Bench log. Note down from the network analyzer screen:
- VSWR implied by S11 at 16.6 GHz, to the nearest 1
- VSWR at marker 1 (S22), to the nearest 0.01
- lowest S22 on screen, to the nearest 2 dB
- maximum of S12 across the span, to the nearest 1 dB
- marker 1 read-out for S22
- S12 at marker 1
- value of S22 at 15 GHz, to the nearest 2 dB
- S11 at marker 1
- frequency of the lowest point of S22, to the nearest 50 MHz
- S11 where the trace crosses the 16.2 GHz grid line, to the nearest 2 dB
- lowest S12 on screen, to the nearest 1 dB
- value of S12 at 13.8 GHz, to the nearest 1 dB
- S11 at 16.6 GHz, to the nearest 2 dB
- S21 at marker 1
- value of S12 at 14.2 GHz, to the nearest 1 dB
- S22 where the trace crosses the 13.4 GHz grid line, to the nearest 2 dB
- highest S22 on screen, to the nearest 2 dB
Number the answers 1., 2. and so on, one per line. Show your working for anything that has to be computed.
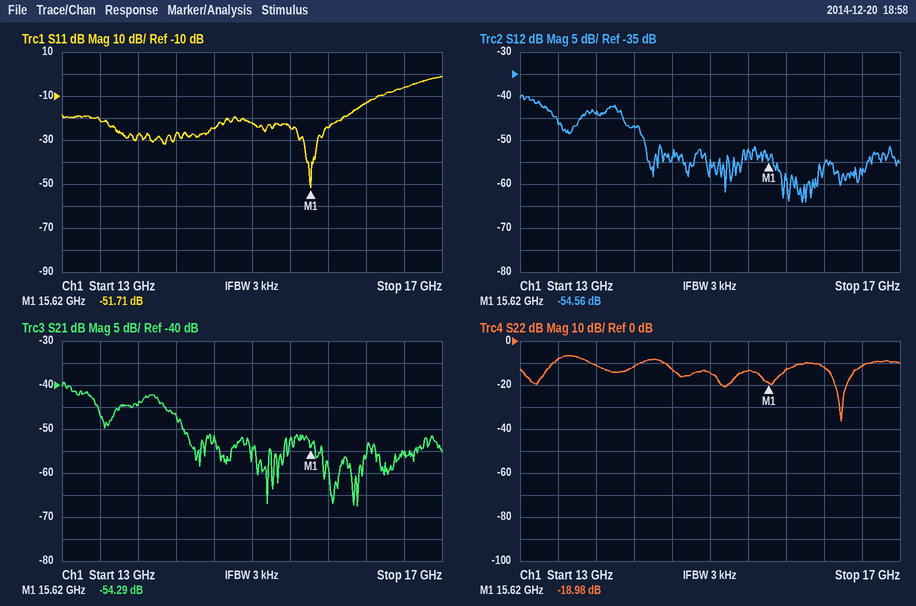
1. |Γ| = 10^(-6/20) = 0.5012; VSWR = (1 + 0.5012)/(1 − 0.5012) ≈ 3
2. (1 + 0.1125)/(1 − 0.1125) ≈ 1.25
3. -36 dB
4. -40 dB
5. -18.98 dB
6. -54.56 dB
7. -14 dB
8. -51.71 dB
9. 16.40 GHz
10. -14 dB
11. -64 dB
12. -44 dB
13. -6 dB
14. -54.29 dB
15. -47 dB
16. -8 dB
17. -6 dB
